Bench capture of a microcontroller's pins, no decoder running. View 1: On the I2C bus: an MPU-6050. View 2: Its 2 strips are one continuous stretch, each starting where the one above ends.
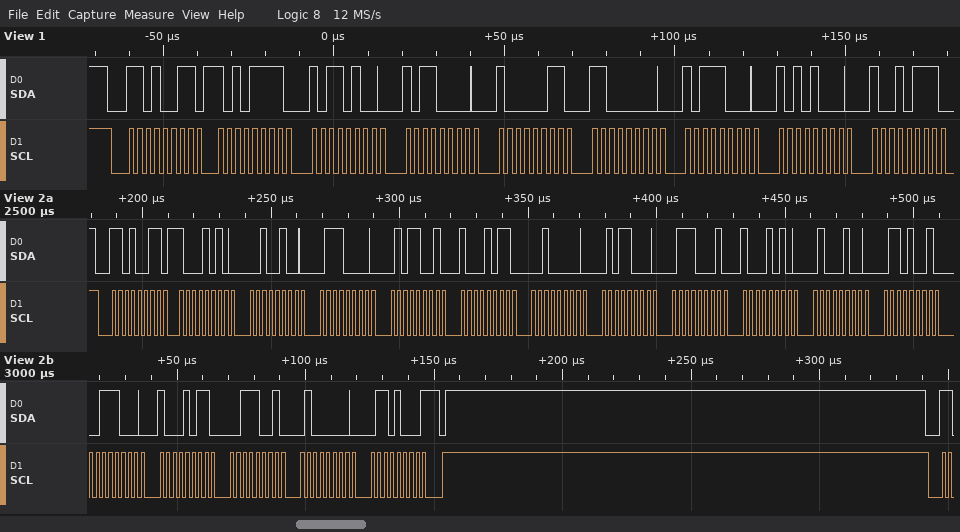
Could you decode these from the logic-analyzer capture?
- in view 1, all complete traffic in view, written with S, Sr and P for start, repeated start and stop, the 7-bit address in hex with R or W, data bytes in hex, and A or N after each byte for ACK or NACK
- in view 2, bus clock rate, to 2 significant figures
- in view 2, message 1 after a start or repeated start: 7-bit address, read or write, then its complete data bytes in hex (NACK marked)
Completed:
S 69R A AF A B4 A B0 A 83 A C0 A B8 A A8 A 97 A
400 kHz
0x69 read: 8A 24 70 59 8B 20 58 71 8A 44 69 38 8B 39 40 68 NACK
